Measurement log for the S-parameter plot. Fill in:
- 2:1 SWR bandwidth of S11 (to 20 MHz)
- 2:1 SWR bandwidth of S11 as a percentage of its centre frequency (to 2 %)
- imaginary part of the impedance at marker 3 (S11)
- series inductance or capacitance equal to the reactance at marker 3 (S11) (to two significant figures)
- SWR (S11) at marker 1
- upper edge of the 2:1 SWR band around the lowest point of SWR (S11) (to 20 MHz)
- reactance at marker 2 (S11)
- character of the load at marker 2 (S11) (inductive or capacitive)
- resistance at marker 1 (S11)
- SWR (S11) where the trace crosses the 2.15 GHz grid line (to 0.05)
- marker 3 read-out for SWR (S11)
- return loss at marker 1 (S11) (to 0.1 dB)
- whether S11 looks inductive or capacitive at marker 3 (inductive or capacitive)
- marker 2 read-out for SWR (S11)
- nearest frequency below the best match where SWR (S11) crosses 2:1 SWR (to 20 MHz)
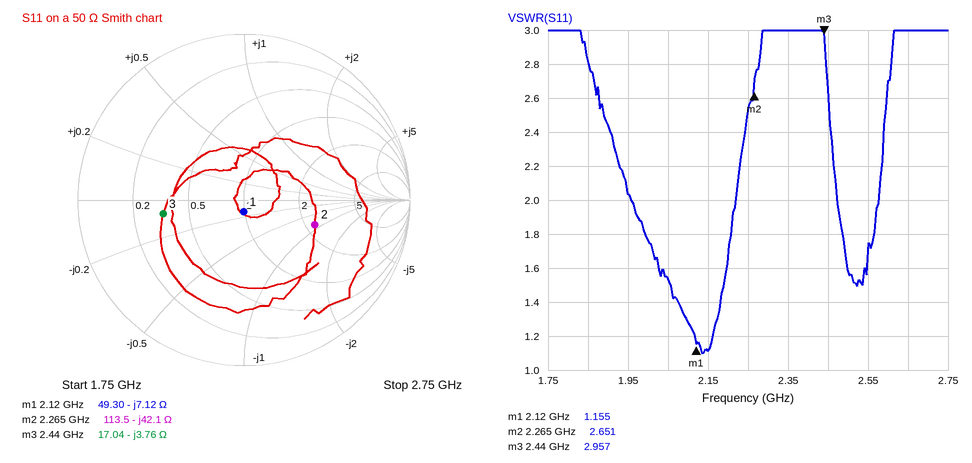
260 MHz
12 %
-3.76 Ω
17 pF
1.155
2.22 GHz
-42.1 Ω
capacitive
49.30 Ω
1.10
2.957
22.9 dB
capacitive
2.651
1.96 GHz
